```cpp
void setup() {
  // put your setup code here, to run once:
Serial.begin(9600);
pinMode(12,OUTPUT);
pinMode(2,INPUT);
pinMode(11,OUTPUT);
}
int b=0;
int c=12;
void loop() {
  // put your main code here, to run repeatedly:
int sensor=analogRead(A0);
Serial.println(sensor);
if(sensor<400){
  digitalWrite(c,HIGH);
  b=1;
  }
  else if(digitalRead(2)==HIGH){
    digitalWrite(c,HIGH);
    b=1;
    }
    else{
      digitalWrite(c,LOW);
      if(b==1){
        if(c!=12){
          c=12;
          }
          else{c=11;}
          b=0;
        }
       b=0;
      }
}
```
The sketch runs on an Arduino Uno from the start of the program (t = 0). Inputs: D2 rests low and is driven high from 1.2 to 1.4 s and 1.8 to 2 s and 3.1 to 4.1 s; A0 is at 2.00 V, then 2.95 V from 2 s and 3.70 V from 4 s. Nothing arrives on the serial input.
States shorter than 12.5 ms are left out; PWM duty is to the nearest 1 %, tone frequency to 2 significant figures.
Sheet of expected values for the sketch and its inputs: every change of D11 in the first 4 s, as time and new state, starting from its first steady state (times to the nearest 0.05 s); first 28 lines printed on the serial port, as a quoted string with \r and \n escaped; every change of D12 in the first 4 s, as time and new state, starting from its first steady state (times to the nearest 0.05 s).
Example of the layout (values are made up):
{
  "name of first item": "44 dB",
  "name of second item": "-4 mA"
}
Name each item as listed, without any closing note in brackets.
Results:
{
  "every change of D11 in the first 4 s, as time and new state, starting from its first steady state": "0 s low; 1.8 s high; 2 s low",
  "first 28 lines printed on the serial port, as a quoted string with \\r and \\n escaped": "\"409\\r\\n409\\r\\n409\\r\\n409\\r\\n409\\r\\n409\\r\\n409\\r\\n409\\r\\n409\\r\\n409\\r\\n409\\r\\n409\\r\\n409\\r\\n409\\r\\n409\\r\\n409\\r\\n409\\r\\n409\\r\\n409\\r\\n409\\r\\n409\\r\\n409\\r\\n409\\r\\n409\\r\\n409\\r\\n409\\r\\n409\\r\\n409\\r\\n\"",
  "every change of D12 in the first 4 s, as time and new state, starting from its first steady state": "0 s low; 1.2 s high; 1.4 s low; 3.1 s high"
}
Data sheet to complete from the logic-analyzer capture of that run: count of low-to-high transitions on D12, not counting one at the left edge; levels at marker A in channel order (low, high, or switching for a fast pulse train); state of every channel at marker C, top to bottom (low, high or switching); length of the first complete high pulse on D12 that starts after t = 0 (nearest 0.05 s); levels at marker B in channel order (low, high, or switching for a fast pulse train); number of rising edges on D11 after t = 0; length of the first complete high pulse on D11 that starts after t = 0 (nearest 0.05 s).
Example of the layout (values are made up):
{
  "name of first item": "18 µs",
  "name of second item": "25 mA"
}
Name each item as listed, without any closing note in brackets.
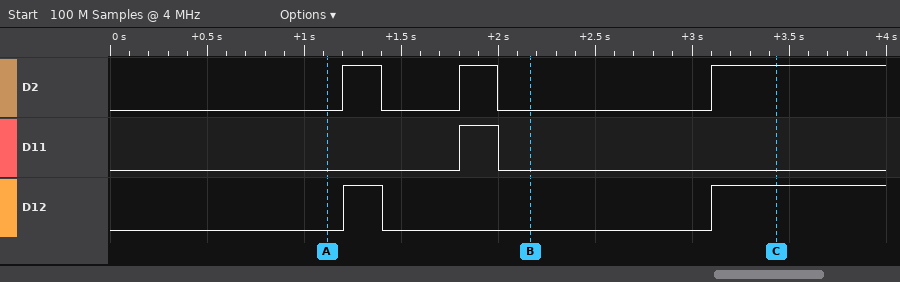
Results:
{
  "count of low-to-high transitions on D12, not counting one at the left edge": "2",
  "levels at marker A in channel order": "D2 low, D11 low, D12 low",
  "state of every channel at marker C, top to bottom": "D2 high, D11 low, D12 high",
  "length of the first complete high pulse on D12 that starts after t = 0": "0.20 s",
  "levels at marker B in channel order": "D2 low, D11 low, D12 low",
  "number of rising edges on D11 after t = 0": "1",
  "length of the first complete high pulse on D11 that starts after t = 0": "0.20 s"
}
